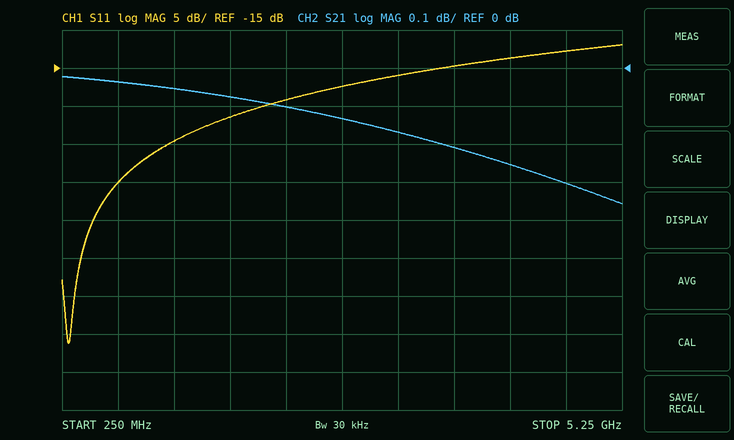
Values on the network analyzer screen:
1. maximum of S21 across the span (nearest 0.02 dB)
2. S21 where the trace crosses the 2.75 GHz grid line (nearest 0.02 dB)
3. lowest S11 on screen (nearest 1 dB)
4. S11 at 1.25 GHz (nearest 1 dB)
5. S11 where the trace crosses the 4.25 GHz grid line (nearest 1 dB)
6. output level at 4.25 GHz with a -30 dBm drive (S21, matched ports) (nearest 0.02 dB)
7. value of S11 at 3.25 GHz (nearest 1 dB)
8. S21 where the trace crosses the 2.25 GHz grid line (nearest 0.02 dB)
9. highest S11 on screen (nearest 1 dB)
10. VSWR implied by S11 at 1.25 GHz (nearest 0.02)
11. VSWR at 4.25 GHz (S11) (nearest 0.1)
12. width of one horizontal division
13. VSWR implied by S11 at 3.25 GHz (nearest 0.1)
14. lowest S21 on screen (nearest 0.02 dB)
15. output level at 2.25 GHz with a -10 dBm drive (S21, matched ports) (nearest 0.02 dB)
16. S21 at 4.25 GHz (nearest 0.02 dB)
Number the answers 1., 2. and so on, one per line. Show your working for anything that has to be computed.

1. -0.02 dB
2. -0.14 dB
3. -51 dB
4. -25 dB
5. -14 dB
6. -30 dBm + (-0.26 dB) = -30.26 dBm
7. -16 dB
8. -0.10 dB
9. -12 dB
10. |Γ| = 10^(-25/20) = 0.0562; VSWR = (1 + 0.0562)/(1 − 0.0562) ≈ 1.12
11. |Γ| = 10^(-14/20) = 0.1995; VSWR = (1 + 0.1995)/(1 − 0.1995) ≈ 1.5
12. 500 MHz
13. |Γ| = 10^(-16/20) = 0.1585; VSWR = (1 + 0.1585)/(1 − 0.1585) ≈ 1.4
14. -0.36 dB
15. -10 dBm + (-0.10 dB) = -10.10 dBm
16. -0.26 dB
